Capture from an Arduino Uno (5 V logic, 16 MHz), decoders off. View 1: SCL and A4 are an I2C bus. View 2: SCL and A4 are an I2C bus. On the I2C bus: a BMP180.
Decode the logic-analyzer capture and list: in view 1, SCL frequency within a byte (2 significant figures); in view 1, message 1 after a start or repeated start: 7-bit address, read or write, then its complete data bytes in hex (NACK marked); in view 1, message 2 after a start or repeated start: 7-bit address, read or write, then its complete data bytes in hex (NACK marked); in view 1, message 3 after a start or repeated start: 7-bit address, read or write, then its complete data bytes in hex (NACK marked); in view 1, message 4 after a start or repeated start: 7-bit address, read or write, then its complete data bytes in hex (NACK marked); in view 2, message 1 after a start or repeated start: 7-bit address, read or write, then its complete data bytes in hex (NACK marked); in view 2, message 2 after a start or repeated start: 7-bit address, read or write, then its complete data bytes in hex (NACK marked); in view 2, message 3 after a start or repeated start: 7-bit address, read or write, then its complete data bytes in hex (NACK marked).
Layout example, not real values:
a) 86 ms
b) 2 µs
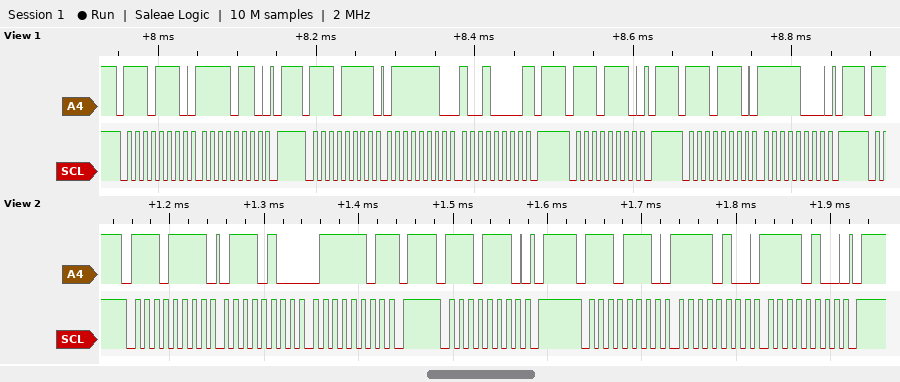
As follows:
a) 100 kHz
b) 0x77 write: F6
c) 0x77 read: 7E 90 NACK
d) 0x77 write
e) 0x77 write: F8
f) 0x77 read: 74 7D NACK
g) 0x77 write
h) 0x77 write: F4 F4
